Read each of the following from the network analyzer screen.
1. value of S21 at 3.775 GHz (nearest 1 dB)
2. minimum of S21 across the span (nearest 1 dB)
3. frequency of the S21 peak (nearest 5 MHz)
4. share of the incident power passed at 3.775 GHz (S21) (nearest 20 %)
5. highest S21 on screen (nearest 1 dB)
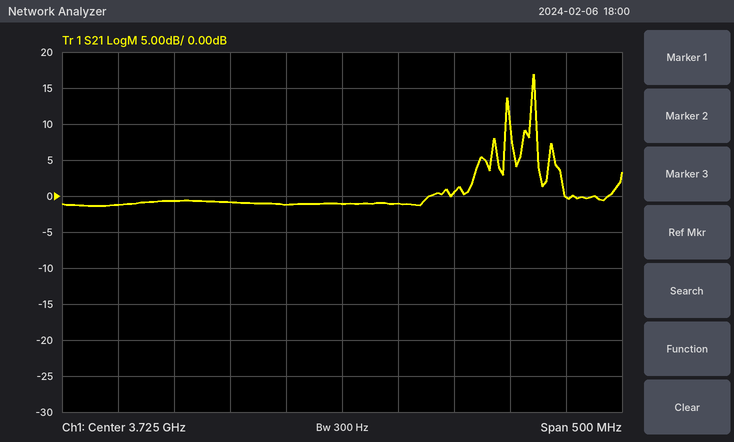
-1 dB
-1 dB
3.895 GHz
80 %
17 dB
